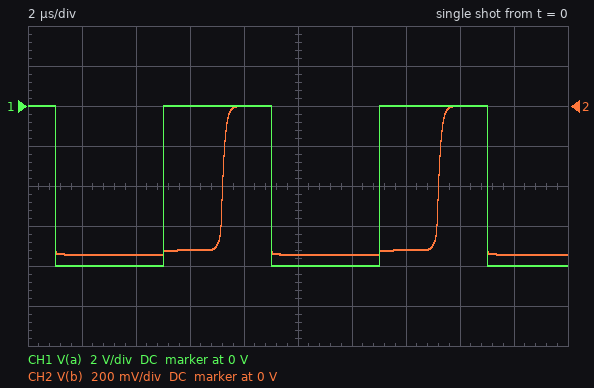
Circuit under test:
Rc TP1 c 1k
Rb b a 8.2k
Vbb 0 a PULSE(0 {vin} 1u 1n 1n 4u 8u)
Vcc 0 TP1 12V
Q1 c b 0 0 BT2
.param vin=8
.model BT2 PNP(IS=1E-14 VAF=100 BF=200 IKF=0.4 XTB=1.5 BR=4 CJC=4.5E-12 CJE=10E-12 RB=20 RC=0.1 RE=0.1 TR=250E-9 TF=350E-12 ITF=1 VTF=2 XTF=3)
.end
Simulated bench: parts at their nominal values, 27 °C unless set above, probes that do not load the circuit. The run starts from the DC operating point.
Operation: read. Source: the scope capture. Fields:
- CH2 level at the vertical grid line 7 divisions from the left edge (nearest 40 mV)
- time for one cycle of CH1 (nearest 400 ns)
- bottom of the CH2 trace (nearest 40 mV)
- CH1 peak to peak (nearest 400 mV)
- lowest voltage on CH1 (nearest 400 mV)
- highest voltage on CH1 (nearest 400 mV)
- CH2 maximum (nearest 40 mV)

-720 mV
8.0 µs
-760 mV
8.0 V
-8.0 V
0 V
0 V
